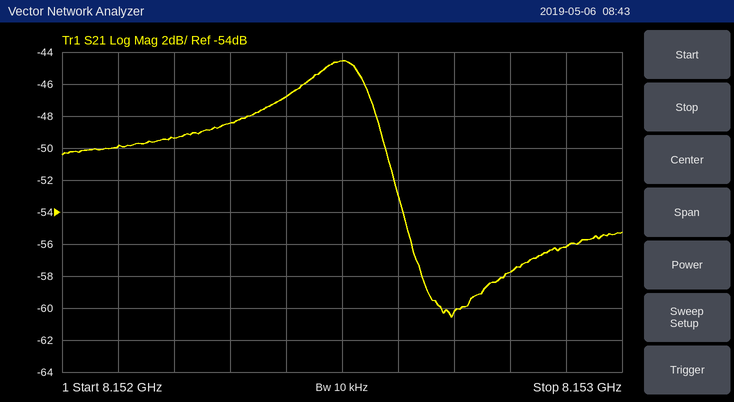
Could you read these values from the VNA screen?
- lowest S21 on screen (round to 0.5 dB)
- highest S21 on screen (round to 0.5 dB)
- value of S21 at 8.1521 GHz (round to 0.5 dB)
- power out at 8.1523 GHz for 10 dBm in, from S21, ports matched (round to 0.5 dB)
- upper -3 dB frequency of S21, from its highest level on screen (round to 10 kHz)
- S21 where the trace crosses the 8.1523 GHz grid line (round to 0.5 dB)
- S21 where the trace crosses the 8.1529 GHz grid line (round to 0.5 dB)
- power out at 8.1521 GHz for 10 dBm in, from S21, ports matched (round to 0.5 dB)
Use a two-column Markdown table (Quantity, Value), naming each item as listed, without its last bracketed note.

| Quantity | Value |
|---|---|
| lowest S21 on screen | -60.5 dB |
| highest S21 on screen | -44.5 dB |
| value of S21 at 8.1521 GHz | -50.0 dB |
| power out at 8.1523 GHz for 10 dBm in, from S21, ports matched | -38.5 dBm |
| upper -3 dB frequency of S21, from its highest level on screen | 8.15256 GHz |
| S21 where the trace crosses the 8.1523 GHz grid line | -48.5 dB |
| S21 where the trace crosses the 8.1529 GHz grid line | -56.0 dB |
| power out at 8.1521 GHz for 10 dBm in, from S21, ports matched | -40.0 dBm |
